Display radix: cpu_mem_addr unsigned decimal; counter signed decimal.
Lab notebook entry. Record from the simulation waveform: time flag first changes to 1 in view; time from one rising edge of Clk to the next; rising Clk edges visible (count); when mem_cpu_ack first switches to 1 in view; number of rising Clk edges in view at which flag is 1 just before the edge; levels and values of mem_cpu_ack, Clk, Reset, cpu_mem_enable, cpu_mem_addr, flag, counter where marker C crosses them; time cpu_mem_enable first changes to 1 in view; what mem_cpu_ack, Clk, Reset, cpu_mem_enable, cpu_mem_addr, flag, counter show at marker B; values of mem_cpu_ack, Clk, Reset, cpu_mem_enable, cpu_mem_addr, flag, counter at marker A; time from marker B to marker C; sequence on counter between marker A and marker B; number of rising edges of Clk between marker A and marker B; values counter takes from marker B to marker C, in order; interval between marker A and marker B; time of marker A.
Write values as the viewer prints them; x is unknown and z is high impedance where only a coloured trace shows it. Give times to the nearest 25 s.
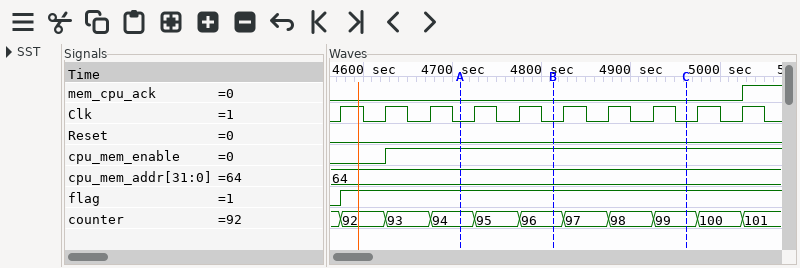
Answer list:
4575 s
50 s
10
5025 s
9
mem_cpu_ack=0, Clk=0, Reset=0, cpu_mem_enable=1, cpu_mem_addr=64, flag=1, counter=99
4625 s
mem_cpu_ack=0, Clk=0, Reset=0, cpu_mem_enable=1, cpu_mem_addr=64, flag=1, counter=96
mem_cpu_ack=0, Clk=0, Reset=0, cpu_mem_enable=1, cpu_mem_addr=64, flag=1, counter=94
150 s
94, 95, 96
2
96, 97, 98, 99
100 s
4700 s
